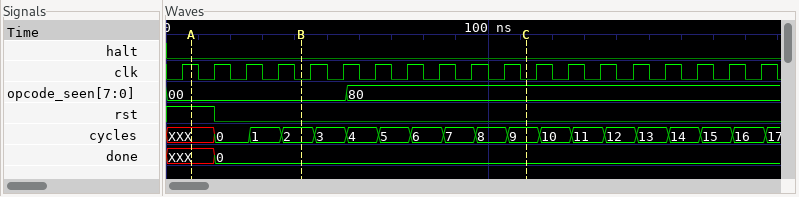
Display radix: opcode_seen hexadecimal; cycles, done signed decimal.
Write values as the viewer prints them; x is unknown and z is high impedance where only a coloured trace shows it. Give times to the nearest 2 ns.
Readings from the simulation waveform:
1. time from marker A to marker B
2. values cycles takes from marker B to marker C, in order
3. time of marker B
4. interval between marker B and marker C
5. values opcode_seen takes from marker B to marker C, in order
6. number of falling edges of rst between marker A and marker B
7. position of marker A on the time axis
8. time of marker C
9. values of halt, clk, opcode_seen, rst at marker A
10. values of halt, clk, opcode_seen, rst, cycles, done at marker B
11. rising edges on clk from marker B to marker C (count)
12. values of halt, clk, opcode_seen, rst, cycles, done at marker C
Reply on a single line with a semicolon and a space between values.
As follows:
34 ns; 2, 3, 4, 5, 6, 7, 8, 9; 42 ns; 70 ns; 00, 80; 1; 8 ns; 112 ns; halt=0, clk=1, opcode_seen=00, rst=1; halt=0, clk=0, opcode_seen=00, rst=0, cycles=2, done=0; 7; halt=0, clk=0, opcode_seen=80, rst=0, cycles=9, done=0
